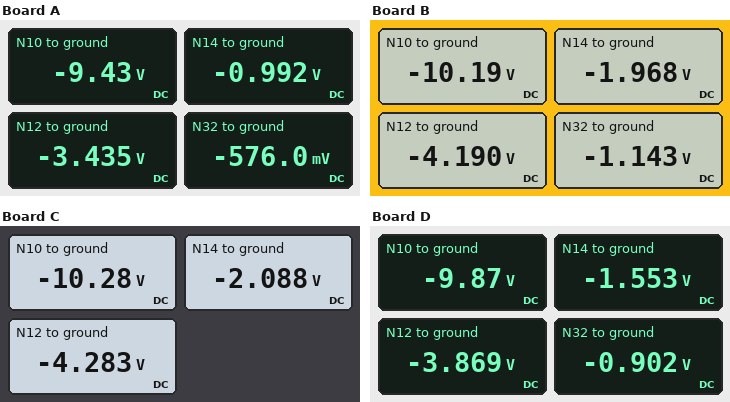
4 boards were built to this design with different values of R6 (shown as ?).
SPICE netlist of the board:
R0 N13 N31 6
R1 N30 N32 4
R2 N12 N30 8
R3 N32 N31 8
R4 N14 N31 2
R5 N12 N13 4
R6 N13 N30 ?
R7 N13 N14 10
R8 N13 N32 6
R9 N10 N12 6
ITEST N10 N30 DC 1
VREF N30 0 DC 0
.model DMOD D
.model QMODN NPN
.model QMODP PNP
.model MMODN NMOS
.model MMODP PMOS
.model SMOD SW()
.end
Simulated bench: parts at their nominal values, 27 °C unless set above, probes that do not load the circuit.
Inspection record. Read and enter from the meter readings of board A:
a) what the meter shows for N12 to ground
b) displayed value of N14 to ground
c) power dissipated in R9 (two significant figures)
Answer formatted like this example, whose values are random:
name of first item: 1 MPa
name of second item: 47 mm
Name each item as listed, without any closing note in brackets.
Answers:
what the meter shows for N12 to ground: -3.435 V
displayed value of N14 to ground: -0.992 V
power dissipated in R9: 6.0 W
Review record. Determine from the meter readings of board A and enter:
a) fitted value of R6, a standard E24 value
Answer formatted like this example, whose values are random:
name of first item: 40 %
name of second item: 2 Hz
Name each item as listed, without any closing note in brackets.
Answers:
fitted value of R6, a standard E24 value: 2.7 Ω
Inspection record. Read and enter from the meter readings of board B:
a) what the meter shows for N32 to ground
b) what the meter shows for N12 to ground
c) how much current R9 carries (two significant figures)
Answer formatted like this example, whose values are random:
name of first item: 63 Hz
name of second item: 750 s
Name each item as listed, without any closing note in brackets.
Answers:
what the meter shows for N32 to ground: -1.143 V
what the meter shows for N12 to ground: -4.190 V
how much current R9 carries: 1.0 A
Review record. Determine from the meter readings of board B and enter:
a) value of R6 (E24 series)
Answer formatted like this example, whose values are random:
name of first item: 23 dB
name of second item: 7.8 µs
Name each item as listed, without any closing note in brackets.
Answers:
value of R6: 12 Ω
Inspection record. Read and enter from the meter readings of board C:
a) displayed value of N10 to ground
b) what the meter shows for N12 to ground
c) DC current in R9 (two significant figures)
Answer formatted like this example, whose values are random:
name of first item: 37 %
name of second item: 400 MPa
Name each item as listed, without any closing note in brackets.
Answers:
displayed value of N10 to ground: -10.28 V
what the meter shows for N12 to ground: -4.283 V
DC current in R9: 1.0 A
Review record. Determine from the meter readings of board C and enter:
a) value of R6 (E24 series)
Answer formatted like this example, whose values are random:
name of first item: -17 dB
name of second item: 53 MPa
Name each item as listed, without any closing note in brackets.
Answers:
value of R6: 15 Ω
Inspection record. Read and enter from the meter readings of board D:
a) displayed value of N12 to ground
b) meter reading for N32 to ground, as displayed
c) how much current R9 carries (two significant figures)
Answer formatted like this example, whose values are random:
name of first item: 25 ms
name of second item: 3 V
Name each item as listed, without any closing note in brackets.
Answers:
displayed value of N12 to ground: -3.869 V
meter reading for N32 to ground, as displayed: -0.902 V
how much current R9 carries: 1.0 A
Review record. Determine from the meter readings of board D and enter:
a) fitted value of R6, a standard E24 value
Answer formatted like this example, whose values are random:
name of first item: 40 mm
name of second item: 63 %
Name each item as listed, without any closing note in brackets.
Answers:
fitted value of R6, a standard E24 value: 6.2 Ω
